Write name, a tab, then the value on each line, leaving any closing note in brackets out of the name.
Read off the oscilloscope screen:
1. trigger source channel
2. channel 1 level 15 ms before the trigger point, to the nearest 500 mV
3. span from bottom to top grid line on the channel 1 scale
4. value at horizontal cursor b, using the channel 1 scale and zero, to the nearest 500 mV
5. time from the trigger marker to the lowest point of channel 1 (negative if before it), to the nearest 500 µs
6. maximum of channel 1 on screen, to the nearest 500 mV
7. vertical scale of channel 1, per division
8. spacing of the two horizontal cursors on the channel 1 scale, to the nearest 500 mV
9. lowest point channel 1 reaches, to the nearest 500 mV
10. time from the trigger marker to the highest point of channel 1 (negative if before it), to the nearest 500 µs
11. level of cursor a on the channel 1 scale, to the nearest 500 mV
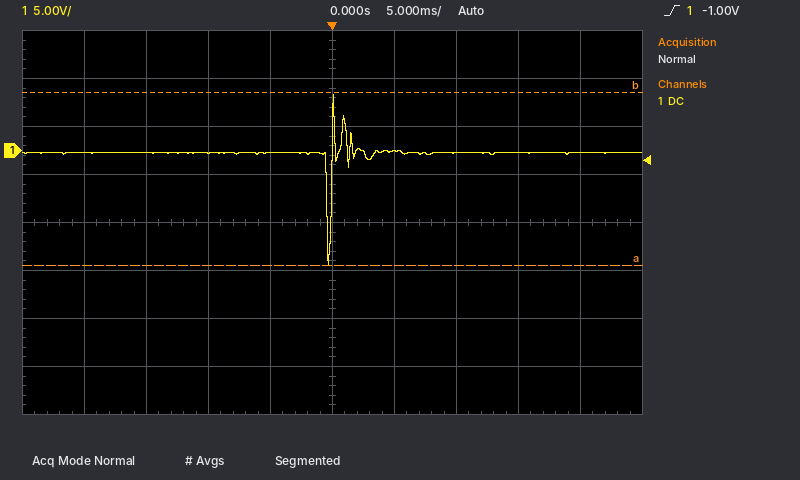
trigger source channel	channel 1
channel 1 level 15 ms before the trigger point, to the nearest 500 mV	0.0 V
span from bottom to top grid line on the channel 1 scale	40 V
value at horizontal cursor b, using the channel 1 scale and zero, to the nearest 500 mV	6.0 V
time from the trigger marker to the lowest point of channel 1 (negative if before it), to the nearest 500 µs	-500 µs
maximum of channel 1 on screen, to the nearest 500 mV	6.0 V
vertical scale of channel 1, per division	5 V
spacing of the two horizontal cursors on the channel 1 scale, to the nearest 500 mV	18.0 V
lowest point channel 1 reaches, to the nearest 500 mV	-12.0 V
time from the trigger marker to the highest point of channel 1 (negative if before it), to the nearest 500 µs	0.0 ms
level of cursor a on the channel 1 scale, to the nearest 500 mV	-12.0 V
